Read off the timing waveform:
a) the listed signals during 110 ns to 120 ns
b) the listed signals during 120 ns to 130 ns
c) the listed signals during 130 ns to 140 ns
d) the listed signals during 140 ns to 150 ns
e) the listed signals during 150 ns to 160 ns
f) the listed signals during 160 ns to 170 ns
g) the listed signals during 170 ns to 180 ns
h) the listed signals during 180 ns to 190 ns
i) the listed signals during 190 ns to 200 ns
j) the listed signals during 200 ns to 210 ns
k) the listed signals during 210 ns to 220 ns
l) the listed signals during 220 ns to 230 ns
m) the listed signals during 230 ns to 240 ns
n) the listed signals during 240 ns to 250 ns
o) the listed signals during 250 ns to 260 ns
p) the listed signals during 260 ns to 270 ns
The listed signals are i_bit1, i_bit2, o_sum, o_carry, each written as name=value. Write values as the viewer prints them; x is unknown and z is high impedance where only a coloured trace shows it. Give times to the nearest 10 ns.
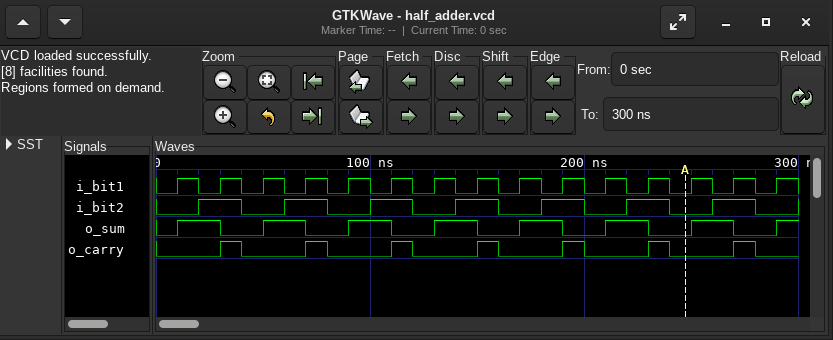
i_bit1=1, i_bit2=1, o_sum=0, o_carry=1
i_bit1=0, i_bit2=0, o_sum=0, o_carry=0
i_bit1=1, i_bit2=0, o_sum=1, o_carry=0
i_bit1=0, i_bit2=1, o_sum=1, o_carry=0
i_bit1=1, i_bit2=1, o_sum=0, o_carry=1
i_bit1=0, i_bit2=0, o_sum=0, o_carry=0
i_bit1=1, i_bit2=0, o_sum=1, o_carry=0
i_bit1=0, i_bit2=1, o_sum=1, o_carry=0
i_bit1=1, i_bit2=1, o_sum=0, o_carry=1
i_bit1=0, i_bit2=0, o_sum=0, o_carry=0
i_bit1=1, i_bit2=0, o_sum=1, o_carry=0
i_bit1=0, i_bit2=1, o_sum=1, o_carry=0
i_bit1=1, i_bit2=1, o_sum=0, o_carry=1
i_bit1=0, i_bit2=0, o_sum=0, o_carry=0
i_bit1=1, i_bit2=0, o_sum=1, o_carry=0
i_bit1=0, i_bit2=1, o_sum=1, o_carry=0
